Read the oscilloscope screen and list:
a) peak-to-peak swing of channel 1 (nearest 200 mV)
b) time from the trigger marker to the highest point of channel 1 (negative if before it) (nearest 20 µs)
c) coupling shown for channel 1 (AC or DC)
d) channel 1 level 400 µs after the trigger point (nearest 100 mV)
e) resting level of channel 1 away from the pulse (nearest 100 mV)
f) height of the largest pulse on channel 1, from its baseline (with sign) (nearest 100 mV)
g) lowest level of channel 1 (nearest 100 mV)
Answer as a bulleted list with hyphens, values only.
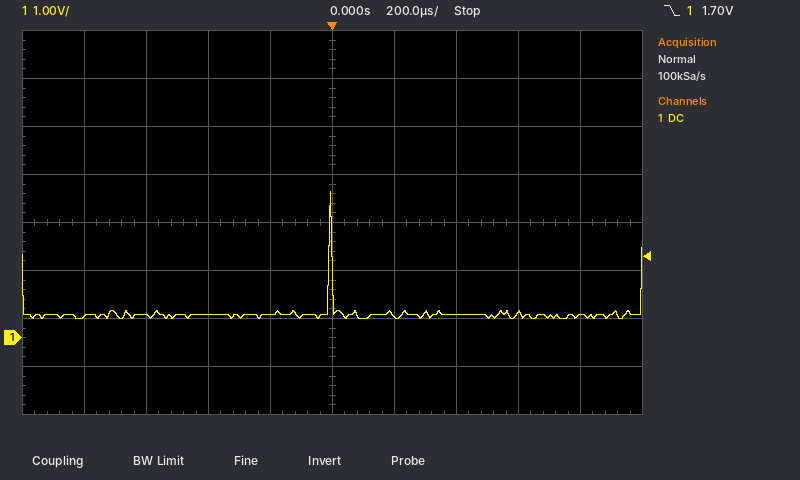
- 2.6 V
- 0 µs
- DC
- 500 mV
- 500 mV
- +2.6 V
- 400 mV
